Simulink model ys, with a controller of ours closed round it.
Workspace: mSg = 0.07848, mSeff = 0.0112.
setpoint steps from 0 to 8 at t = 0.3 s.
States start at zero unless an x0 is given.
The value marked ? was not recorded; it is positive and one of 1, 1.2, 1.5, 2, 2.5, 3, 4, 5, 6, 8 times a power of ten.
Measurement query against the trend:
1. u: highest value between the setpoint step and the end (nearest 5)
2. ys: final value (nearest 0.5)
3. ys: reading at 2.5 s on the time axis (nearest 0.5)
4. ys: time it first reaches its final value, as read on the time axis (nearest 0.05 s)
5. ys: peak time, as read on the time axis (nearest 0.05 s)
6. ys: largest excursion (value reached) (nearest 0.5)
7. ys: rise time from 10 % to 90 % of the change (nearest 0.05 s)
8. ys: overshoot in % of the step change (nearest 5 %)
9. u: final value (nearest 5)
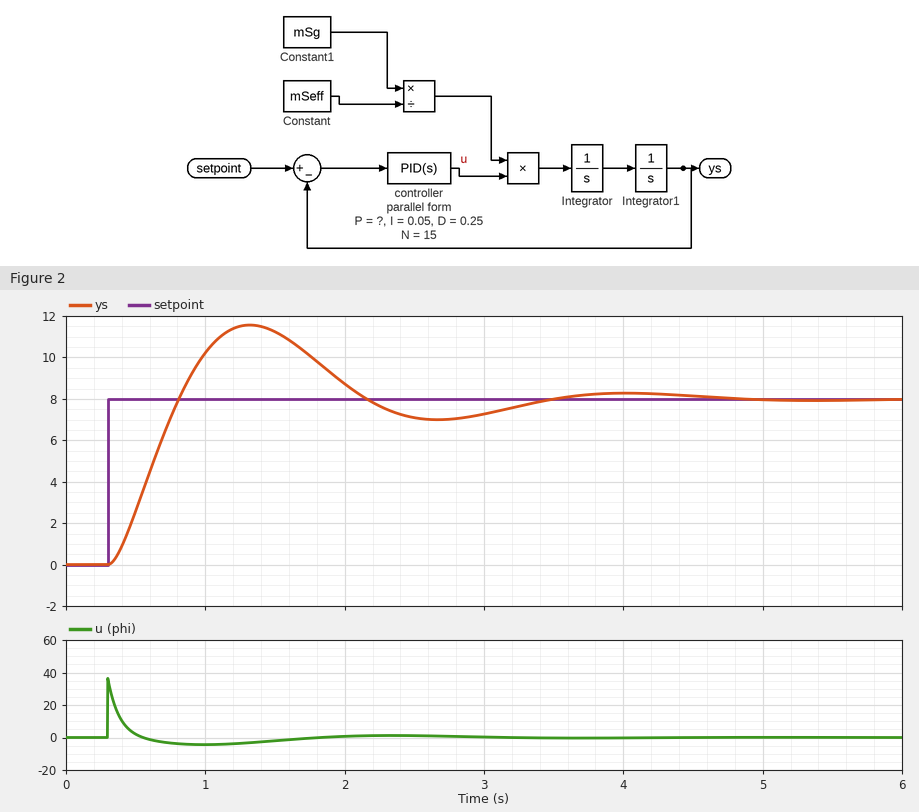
35
8.0
7.0
0.80 s
1.30 s
11.5
0.35 s
45 %
0
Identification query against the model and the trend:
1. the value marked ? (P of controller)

0.8
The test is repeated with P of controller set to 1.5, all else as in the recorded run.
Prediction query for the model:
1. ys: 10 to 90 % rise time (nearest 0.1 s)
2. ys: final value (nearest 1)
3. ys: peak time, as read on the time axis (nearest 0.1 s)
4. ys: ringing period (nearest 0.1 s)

0.3 s
8
1.1 s
1.9 s
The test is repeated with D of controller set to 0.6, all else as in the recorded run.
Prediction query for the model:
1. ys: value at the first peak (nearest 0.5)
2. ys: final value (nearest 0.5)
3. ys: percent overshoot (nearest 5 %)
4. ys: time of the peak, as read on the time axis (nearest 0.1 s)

9.5
8.0
20 %
1.0 s
